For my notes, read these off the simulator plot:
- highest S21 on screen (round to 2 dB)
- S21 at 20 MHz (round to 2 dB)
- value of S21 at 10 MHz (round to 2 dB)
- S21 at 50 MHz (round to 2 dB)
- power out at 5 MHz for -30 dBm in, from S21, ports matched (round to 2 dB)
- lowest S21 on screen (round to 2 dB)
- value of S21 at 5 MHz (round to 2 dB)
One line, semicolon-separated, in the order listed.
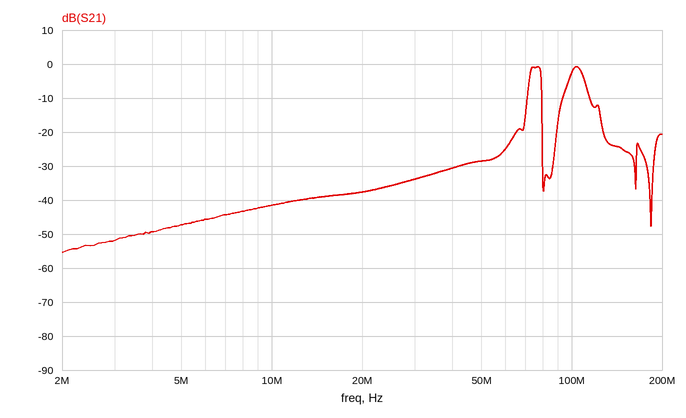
0 dB; -38 dB; -42 dB; -28 dB; -78 dBm; -56 dB; -48 dB
